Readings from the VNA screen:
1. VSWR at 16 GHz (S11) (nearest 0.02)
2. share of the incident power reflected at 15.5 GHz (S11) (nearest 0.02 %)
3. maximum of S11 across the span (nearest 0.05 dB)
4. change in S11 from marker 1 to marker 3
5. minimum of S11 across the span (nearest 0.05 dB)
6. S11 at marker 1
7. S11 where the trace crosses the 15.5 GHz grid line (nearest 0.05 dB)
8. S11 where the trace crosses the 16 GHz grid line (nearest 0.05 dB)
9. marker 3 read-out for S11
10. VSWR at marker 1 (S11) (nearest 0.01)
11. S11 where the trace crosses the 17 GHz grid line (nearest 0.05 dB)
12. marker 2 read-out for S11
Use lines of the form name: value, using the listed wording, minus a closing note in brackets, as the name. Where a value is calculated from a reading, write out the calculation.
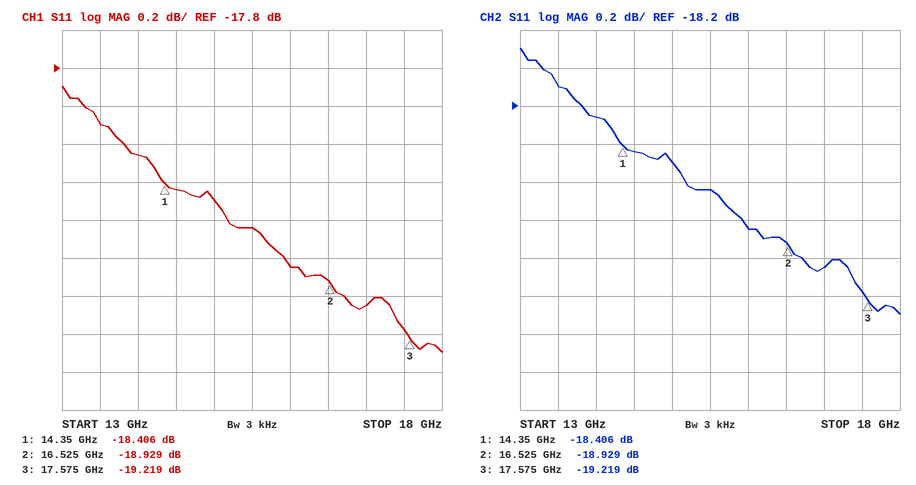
VSWR at 16 GHz (S11): |Γ| = 10^(-18.85/20) = 0.1142; VSWR = (1 + 0.1142)/(1 − 0.1142) ≈ 1.26
share of the incident power reflected at 15.5 GHz (S11): 10^(-18.65/10) ≈ 1.36 %
maximum of S11 across the span: -17.90 dB
change in S11 from marker 1 to marker 3: -19.219 − (-18.406) = -0.813 dB
minimum of S11 across the span: -19.30 dB
S11 at marker 1: -18.406 dB
S11 where the trace crosses the 15.5 GHz grid line: -18.65 dB
S11 where the trace crosses the 16 GHz grid line: -18.85 dB
marker 3 read-out for S11: -19.219 dB
VSWR at marker 1 (S11): (1 + 0.1201)/(1 − 0.1201) ≈ 1.27
S11 where the trace crosses the 17 GHz grid line: -19.05 dB
marker 2 read-out for S11: -18.929 dB
